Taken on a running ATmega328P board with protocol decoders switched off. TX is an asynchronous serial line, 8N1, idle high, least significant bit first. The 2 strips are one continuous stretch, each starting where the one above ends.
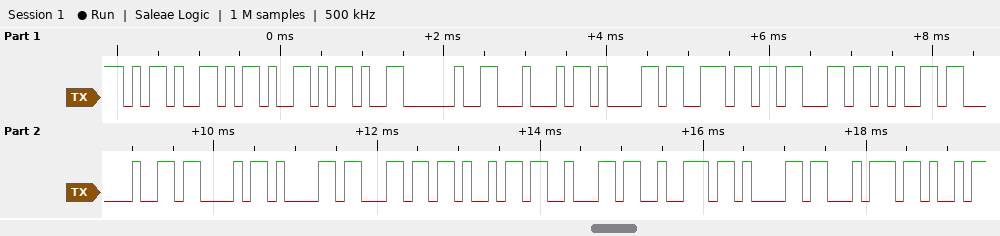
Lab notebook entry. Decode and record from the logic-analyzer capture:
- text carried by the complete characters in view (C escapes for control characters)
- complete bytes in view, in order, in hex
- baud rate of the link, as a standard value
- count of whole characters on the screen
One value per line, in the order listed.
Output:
"--- Dance Calibrat"
2D 2D 2D 20 44 61 6E 63 65 20 43 61 6C 69 62 72 61 74
9600 baud
18
